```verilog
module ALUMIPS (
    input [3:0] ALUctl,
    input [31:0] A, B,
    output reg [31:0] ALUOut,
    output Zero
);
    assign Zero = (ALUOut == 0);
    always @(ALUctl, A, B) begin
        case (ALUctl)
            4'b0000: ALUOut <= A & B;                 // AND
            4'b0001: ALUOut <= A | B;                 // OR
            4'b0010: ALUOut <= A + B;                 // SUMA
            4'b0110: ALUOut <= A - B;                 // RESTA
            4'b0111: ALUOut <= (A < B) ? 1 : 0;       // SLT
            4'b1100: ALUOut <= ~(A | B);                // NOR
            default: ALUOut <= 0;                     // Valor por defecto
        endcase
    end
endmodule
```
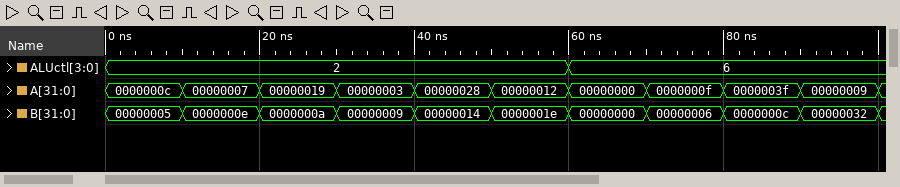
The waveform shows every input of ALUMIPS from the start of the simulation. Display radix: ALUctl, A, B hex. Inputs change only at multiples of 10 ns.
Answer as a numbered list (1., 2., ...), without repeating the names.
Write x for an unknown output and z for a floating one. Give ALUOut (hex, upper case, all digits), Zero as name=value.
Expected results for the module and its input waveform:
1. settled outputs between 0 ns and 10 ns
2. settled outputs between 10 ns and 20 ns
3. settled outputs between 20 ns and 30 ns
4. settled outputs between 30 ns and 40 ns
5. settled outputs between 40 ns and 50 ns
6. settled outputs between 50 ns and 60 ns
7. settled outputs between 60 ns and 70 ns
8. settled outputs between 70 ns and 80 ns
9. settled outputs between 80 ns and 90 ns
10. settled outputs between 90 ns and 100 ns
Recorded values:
1. ALUOut=00000011, Zero=0
2. ALUOut=00000015, Zero=0
3. ALUOut=00000023, Zero=0
4. ALUOut=0000000C, Zero=0
5. ALUOut=0000003C, Zero=0
6. ALUOut=00000030, Zero=0
7. ALUOut=00000000, Zero=1
8. ALUOut=00000009, Zero=0
9. ALUOut=00000033, Zero=0
10. ALUOut=FFFFFFD7, Zero=0
